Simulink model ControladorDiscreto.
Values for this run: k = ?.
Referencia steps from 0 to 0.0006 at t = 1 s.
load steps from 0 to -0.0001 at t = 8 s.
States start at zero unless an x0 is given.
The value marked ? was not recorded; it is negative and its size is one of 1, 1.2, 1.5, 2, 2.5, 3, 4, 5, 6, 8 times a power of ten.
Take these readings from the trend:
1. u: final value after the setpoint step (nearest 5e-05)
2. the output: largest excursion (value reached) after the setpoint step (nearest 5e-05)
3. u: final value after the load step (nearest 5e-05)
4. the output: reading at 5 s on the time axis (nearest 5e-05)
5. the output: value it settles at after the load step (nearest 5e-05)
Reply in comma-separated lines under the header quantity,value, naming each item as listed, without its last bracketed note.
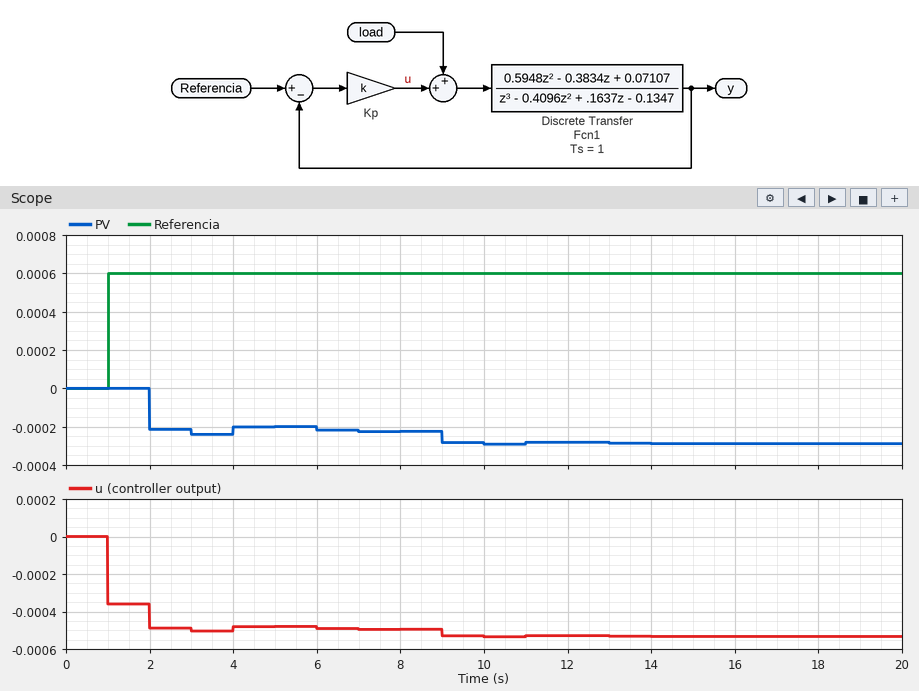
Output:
quantity,value
u: final value after the setpoint step,-0.00050
the output: largest excursion (value reached) after the setpoint step,-0.00025
u: final value after the load step,-0.00055
the output: reading at 5 s on the time axis,-0.00020
the output: value it settles at after the load step,-0.00030
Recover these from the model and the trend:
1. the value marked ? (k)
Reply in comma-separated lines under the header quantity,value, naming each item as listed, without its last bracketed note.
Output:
quantity,value
the value marked ?,-0.6
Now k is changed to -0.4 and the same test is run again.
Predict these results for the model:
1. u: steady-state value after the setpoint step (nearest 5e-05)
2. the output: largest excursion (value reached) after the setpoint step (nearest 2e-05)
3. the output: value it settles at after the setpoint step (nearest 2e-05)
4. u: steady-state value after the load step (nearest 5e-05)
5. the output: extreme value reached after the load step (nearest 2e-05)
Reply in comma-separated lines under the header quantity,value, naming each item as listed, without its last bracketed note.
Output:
quantity,value
u: steady-state value after the setpoint step,-0.00030
the output: largest excursion (value reached) after the setpoint step,-0.00014
the output: value it settles at after the setpoint step,-0.00014
u: steady-state value after the load step,-0.00030
the output: extreme value reached after the load step,-0.00020
